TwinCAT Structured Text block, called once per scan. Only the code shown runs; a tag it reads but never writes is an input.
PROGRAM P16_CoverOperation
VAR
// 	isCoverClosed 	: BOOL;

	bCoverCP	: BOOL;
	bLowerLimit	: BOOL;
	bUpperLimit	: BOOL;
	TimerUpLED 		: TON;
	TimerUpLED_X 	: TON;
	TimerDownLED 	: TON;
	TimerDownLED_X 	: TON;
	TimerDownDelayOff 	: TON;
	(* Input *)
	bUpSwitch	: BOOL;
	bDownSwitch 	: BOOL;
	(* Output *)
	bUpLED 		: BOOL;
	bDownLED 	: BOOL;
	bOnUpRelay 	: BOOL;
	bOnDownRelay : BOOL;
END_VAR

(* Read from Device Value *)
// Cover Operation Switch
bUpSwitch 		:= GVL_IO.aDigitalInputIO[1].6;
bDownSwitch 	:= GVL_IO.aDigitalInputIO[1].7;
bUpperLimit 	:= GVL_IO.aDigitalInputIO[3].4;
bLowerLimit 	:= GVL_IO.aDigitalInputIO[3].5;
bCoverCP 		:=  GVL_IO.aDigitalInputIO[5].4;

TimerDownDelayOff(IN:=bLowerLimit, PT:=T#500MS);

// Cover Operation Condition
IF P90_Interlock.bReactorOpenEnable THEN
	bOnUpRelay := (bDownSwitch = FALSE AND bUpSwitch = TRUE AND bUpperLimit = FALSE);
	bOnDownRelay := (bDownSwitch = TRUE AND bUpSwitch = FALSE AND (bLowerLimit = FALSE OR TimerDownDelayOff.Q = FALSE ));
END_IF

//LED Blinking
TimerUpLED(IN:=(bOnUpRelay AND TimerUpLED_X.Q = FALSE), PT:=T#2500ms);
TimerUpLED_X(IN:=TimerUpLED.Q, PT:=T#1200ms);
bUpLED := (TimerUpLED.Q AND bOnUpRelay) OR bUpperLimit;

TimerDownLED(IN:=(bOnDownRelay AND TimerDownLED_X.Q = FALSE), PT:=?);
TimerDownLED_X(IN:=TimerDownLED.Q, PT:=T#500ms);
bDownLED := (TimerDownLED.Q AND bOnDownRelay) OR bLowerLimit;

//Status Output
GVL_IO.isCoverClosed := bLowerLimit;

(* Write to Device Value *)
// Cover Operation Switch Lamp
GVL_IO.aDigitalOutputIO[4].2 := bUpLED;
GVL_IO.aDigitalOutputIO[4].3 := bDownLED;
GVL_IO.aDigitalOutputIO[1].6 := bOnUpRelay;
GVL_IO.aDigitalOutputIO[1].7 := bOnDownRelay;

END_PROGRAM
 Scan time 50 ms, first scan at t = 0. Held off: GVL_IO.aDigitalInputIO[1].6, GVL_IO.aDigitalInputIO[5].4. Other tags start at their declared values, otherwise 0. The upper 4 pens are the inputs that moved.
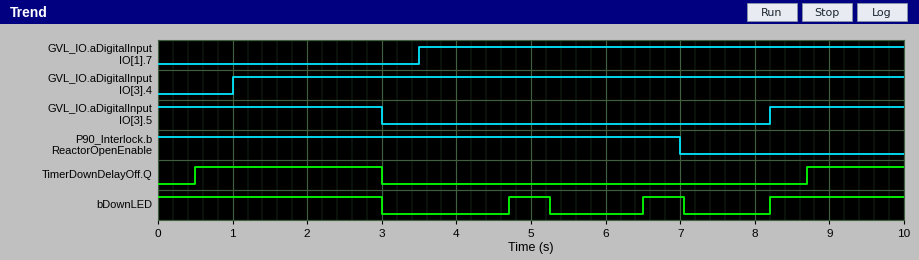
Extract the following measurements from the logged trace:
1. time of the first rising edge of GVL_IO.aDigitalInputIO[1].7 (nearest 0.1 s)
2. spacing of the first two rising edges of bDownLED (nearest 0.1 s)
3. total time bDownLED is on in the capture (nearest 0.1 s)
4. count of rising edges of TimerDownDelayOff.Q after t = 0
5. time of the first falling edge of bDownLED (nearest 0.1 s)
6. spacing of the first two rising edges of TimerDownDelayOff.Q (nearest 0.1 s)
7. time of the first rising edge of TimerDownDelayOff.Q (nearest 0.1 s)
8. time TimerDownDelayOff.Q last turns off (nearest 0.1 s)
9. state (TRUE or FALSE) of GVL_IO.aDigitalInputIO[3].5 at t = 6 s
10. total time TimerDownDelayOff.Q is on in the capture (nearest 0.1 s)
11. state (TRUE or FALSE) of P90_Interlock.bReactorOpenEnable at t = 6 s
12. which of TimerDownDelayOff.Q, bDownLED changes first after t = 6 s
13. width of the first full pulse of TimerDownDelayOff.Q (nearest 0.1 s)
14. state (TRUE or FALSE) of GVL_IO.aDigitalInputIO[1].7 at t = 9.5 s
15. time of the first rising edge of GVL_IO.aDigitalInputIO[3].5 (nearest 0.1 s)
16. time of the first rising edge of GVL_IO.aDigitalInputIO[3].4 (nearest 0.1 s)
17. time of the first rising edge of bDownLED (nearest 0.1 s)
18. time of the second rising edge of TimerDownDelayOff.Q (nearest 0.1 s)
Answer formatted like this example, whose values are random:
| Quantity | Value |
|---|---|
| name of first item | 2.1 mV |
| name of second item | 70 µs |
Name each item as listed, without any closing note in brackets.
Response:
| Quantity | Value |
|---|---|
| time of the first rising edge of GVL_IO.aDigitalInputIO[1].7 | 3.5 s |
| spacing of the first two rising edges of bDownLED | 1.8 s |
| total time bDownLED is on in the capture | 5.9 s |
| count of rising edges of TimerDownDelayOff.Q after t = 0 | 2 |
| time of the first falling edge of bDownLED | 3.0 s |
| spacing of the first two rising edges of TimerDownDelayOff.Q | 8.2 s |
| time of the first rising edge of TimerDownDelayOff.Q | 0.5 s |
| time TimerDownDelayOff.Q last turns off | 3.0 s |
| state (TRUE or FALSE) of GVL_IO.aDigitalInputIO[3].5 at t = 6 s | FALSE |
| total time TimerDownDelayOff.Q is on in the capture | 3.8 s |
| state (TRUE or FALSE) of P90_Interlock.bReactorOpenEnable at t = 6 s | TRUE |
| which of TimerDownDelayOff.Q, bDownLED changes first after t = 6 s | bDownLED |
| width of the first full pulse of TimerDownDelayOff.Q | 2.5 s |
| state (TRUE or FALSE) of GVL_IO.aDigitalInputIO[1].7 at t = 9.5 s | TRUE |
| time of the first rising edge of GVL_IO.aDigitalInputIO[3].5 | 8.2 s |
| time of the first rising edge of GVL_IO.aDigitalInputIO[3].4 | 1.0 s |
| time of the first rising edge of bDownLED | 4.7 s |
| time of the second rising edge of TimerDownDelayOff.Q | 8.7 s |
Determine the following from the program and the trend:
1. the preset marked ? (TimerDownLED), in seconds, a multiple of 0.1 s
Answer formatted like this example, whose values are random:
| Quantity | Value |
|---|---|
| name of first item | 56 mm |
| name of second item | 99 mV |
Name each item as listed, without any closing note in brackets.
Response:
| Quantity | Value |
|---|---|
| the preset marked ? (TimerDownLED), in seconds, a multiple of 0.1 s | 1.2 s |
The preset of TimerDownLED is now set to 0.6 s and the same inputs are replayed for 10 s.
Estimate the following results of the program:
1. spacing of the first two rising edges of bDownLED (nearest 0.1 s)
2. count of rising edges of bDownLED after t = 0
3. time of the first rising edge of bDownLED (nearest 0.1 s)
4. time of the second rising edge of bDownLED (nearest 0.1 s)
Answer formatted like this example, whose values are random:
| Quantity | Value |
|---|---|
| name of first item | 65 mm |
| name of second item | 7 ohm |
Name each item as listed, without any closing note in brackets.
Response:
| Quantity | Value |
|---|---|
| spacing of the first two rising edges of bDownLED | 1.2 s |
| count of rising edges of bDownLED after t = 0 | 4 |
| time of the first rising edge of bDownLED | 4.1 s |
| time of the second rising edge of bDownLED | 5.3 s |
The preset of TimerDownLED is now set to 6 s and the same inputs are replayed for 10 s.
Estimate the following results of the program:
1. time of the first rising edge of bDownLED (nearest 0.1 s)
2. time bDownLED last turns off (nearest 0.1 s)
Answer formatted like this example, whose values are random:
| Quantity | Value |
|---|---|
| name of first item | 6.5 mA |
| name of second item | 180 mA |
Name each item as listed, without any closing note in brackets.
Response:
| Quantity | Value |
|---|---|
| time of the first rising edge of bDownLED | 8.2 s |
| time bDownLED last turns off | 3.0 s |
